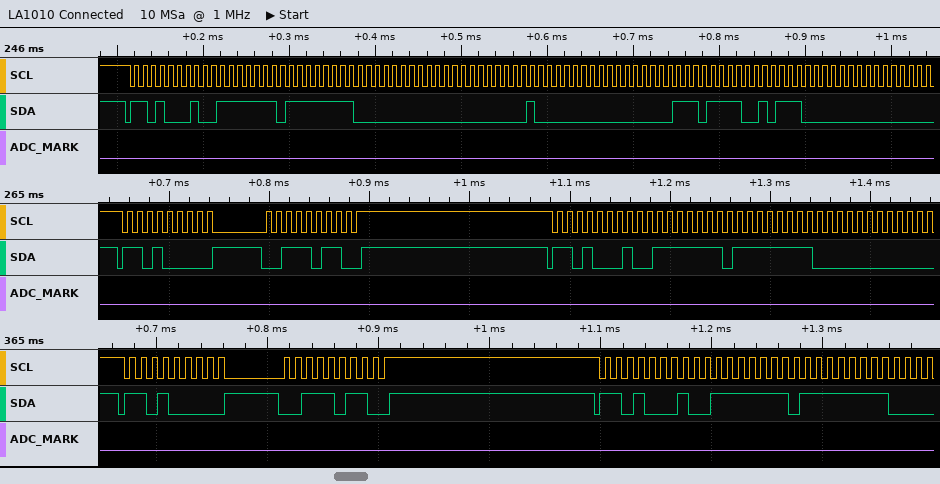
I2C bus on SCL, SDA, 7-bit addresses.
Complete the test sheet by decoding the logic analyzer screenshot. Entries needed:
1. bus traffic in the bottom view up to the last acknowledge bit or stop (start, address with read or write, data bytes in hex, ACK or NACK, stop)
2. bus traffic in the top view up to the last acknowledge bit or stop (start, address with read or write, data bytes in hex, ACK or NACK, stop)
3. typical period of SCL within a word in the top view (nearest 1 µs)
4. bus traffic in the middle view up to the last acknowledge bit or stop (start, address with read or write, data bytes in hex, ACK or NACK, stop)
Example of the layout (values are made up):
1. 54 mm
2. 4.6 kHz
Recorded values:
1. start, address 68 write ACK, 3B ACK, stop, start, address 68 read ACK, 7F ACK, FF ACK
2. start, address 68 read ACK, 7F ACK, FF ACK, 00 ACK, 00 ACK, 40 ACK, 00 ACK, EF ACK, 5C ACK, 00 ACK
3. 10 µs
4. start, address 68 write ACK, 3B ACK, stop, start, address 68 read ACK, 7F ACK, FF ACK, 00 ACK
